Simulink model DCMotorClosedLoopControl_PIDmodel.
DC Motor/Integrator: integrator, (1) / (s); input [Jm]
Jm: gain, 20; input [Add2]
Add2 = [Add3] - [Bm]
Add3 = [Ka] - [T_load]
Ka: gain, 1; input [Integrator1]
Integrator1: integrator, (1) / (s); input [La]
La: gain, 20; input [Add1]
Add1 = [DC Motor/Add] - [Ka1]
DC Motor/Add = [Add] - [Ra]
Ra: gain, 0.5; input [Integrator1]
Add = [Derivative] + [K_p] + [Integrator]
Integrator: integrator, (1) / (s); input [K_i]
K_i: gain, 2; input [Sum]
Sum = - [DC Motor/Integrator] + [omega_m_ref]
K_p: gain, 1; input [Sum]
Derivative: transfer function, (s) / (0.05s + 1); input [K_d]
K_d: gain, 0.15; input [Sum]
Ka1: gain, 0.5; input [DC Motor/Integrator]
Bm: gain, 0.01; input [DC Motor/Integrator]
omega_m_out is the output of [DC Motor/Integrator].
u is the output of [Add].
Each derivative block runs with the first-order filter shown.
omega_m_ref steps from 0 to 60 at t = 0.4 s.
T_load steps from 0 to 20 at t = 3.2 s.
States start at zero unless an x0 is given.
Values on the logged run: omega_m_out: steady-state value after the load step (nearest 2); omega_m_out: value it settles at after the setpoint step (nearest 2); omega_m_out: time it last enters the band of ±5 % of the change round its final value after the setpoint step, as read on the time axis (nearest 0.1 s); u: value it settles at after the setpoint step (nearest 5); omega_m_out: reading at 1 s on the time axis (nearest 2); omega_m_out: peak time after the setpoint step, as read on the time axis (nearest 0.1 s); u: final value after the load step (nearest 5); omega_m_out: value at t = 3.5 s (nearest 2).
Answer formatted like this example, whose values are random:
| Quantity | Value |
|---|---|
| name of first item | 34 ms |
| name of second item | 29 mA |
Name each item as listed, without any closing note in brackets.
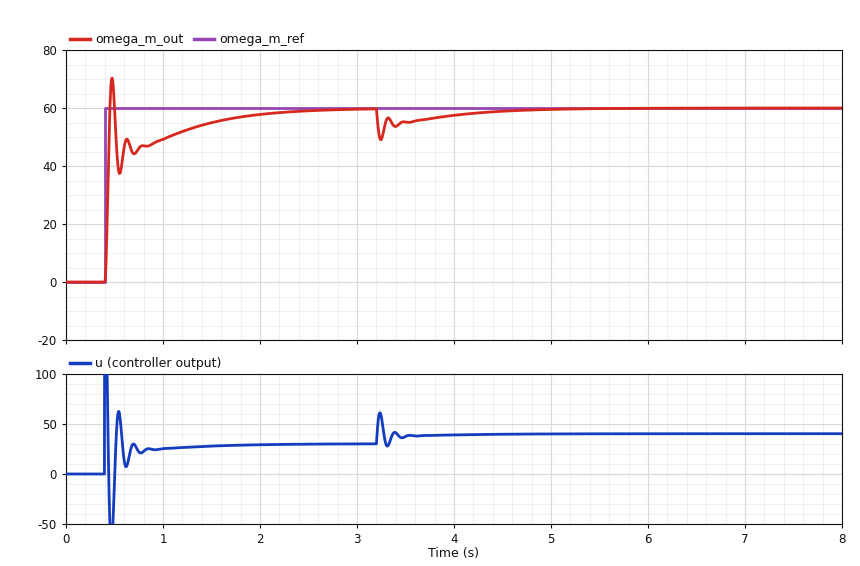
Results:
| Quantity | Value |
|---|---|
| omega_m_out: steady-state value after the load step | 60 |
| omega_m_out: value it settles at after the setpoint step | 60 |
| omega_m_out: time it last enters the band of ±5 % of the change round its final value after the setpoint step, as read on the time axis | 1.8 s |
| u: value it settles at after the setpoint step | 30 |
| omega_m_out: reading at 1 s on the time axis | 50 |
| omega_m_out: peak time after the setpoint step, as read on the time axis | 0.5 s |
| u: final value after the load step | 40 |
| omega_m_out: value at t = 3.5 s | 56 |
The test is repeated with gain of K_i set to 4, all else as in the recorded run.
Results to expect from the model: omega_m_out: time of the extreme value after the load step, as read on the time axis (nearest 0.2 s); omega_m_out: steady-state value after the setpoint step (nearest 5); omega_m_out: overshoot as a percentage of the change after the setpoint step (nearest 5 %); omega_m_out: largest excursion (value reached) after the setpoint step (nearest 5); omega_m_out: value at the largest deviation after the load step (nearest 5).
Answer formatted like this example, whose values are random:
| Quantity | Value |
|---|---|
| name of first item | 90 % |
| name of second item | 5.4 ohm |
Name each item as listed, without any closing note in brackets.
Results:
| Quantity | Value |
|---|---|
| omega_m_out: time of the extreme value after the load step, as read on the time axis | 3.2 s |
| omega_m_out: steady-state value after the setpoint step | 60 |
| omega_m_out: overshoot as a percentage of the change after the setpoint step | 20 % |
| omega_m_out: largest excursion (value reached) after the setpoint step | 70 |
| omega_m_out: value at the largest deviation after the load step | 50 |
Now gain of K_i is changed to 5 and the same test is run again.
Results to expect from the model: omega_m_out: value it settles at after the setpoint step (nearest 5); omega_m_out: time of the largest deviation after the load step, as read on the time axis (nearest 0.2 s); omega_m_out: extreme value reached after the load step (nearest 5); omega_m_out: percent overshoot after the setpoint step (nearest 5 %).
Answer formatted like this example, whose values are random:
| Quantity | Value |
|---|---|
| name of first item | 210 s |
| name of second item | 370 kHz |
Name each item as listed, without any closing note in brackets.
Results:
| Quantity | Value |
|---|---|
| omega_m_out: value it settles at after the setpoint step | 60 |
| omega_m_out: time of the largest deviation after the load step, as read on the time axis | 3.2 s |
| omega_m_out: extreme value reached after the load step | 50 |
| omega_m_out: percent overshoot after the setpoint step | 20 % |
